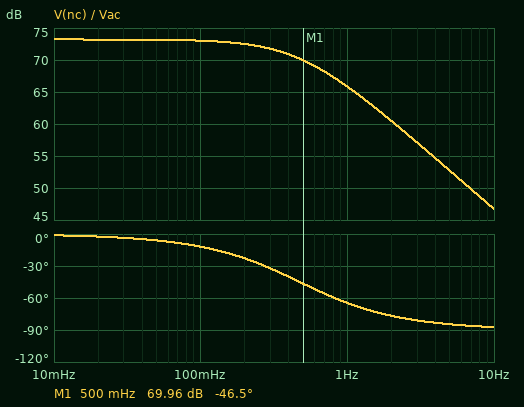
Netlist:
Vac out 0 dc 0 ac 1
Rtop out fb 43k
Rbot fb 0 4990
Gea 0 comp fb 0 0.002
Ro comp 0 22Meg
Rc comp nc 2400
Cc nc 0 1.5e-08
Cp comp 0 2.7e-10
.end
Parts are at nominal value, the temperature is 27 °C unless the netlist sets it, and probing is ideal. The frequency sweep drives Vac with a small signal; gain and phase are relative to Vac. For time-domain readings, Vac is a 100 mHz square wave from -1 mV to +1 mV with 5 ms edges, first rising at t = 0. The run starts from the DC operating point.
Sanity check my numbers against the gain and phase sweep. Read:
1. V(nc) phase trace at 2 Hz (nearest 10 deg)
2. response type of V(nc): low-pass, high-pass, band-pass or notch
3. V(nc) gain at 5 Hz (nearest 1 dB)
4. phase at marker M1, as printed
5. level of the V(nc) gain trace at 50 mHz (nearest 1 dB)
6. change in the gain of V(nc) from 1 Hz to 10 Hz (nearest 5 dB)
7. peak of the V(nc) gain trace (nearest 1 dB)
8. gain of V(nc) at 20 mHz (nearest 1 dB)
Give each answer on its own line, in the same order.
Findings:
-80 deg
low-pass
53 dB
-46.5 deg
73 dB
-20 dB
73 dB
73 dB
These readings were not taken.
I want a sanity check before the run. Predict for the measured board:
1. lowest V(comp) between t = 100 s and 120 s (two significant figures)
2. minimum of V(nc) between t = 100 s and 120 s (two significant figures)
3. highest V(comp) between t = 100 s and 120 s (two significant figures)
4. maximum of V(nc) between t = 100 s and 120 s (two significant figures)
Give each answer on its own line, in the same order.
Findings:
-4.6 V
-4.6 V
4.6 V
4.6 V
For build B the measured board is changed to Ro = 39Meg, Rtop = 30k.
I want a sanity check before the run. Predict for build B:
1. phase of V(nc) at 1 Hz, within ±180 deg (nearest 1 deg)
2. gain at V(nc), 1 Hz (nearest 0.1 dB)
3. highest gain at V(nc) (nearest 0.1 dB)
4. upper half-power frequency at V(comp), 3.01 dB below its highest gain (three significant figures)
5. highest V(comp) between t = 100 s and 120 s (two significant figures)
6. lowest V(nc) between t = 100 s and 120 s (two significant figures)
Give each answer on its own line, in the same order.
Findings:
-75 deg
69.2 dB
80.9 dB
267 mHz
11 V
-11 V
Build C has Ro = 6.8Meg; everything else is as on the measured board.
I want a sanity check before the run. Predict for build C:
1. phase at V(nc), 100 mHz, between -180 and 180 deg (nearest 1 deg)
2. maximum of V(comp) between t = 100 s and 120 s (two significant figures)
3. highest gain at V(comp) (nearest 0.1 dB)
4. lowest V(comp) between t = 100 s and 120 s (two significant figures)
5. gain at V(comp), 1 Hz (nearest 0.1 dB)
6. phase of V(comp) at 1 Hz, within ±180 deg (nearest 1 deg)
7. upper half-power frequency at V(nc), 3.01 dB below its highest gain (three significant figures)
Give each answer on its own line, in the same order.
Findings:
-4 deg
1.4 V
63.0 dB
-1.4 V
61.5 dB
-33 deg
1.53 Hz
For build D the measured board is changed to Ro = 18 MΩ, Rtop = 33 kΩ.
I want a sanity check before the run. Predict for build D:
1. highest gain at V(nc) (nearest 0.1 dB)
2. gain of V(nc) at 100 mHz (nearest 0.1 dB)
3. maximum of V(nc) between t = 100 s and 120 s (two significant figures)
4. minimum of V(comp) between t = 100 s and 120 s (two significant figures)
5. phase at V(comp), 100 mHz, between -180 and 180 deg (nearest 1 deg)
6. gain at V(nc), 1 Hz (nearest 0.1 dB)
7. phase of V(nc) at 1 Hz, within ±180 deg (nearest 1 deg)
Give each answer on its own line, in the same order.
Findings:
73.5 dB
73.4 dB
4.7 V
-4.7 V
-10 deg
67.5 dB
-60 deg
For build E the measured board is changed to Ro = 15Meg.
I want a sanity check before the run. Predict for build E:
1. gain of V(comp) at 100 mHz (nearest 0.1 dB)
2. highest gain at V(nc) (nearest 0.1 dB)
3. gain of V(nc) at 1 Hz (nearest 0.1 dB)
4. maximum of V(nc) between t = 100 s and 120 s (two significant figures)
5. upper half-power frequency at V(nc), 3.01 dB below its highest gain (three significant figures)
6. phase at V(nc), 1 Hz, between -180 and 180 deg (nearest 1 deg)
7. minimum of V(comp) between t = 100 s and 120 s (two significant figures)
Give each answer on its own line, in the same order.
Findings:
69.8 dB
69.9 dB
65.0 dB
3.1 V
695 mHz
-55 deg
-3.1 V
